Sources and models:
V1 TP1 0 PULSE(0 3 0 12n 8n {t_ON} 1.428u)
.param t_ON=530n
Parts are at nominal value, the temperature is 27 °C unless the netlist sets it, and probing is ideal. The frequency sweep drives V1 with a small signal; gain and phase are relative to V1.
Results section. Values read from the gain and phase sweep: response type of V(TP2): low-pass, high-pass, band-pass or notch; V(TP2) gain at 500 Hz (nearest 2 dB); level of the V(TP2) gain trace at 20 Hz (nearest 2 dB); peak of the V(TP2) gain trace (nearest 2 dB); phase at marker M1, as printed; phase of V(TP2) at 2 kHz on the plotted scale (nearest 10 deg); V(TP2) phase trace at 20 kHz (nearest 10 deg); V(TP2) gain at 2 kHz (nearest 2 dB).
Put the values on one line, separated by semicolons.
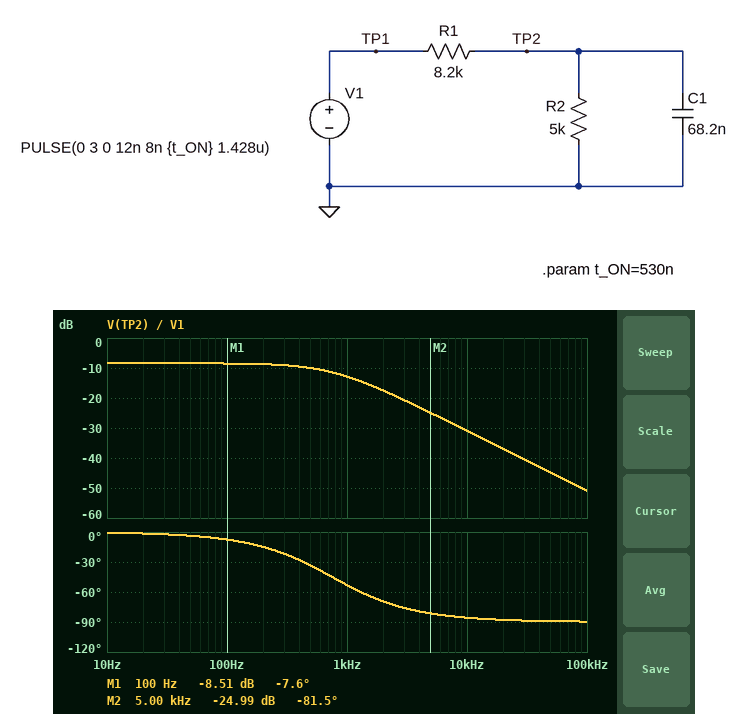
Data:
low-pass; -10 dB; -8 dB; -8 dB; -7.6 deg; -70 deg; -90 deg; -18 dB
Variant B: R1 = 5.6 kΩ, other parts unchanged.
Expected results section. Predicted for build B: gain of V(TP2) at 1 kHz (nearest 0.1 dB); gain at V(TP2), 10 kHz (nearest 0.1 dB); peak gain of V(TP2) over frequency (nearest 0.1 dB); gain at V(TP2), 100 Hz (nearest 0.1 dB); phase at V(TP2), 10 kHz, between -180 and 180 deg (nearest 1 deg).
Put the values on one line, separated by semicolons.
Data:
-10.1 dB; -27.6 dB; -6.5 dB; -6.6 dB; -85 deg
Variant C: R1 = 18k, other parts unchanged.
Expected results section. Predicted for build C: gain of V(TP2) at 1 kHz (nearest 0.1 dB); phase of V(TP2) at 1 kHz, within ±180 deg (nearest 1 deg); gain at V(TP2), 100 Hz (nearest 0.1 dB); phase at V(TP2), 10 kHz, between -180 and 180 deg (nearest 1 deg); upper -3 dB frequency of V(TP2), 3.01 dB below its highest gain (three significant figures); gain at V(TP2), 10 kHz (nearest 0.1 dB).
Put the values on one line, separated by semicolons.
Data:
-19.1 dB; -59 deg; -13.4 dB; -87 deg; 596 Hz; -37.8 dB
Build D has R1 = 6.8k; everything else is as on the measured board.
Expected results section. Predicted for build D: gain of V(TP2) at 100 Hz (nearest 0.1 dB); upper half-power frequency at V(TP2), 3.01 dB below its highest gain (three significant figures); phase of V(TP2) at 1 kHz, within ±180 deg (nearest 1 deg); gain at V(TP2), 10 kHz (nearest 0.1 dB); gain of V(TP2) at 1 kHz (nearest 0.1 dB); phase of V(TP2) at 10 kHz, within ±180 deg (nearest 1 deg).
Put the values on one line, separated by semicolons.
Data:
-7.5 dB; 810 Hz; -51 deg; -29.3 dB; -11.5 dB; -85 deg
